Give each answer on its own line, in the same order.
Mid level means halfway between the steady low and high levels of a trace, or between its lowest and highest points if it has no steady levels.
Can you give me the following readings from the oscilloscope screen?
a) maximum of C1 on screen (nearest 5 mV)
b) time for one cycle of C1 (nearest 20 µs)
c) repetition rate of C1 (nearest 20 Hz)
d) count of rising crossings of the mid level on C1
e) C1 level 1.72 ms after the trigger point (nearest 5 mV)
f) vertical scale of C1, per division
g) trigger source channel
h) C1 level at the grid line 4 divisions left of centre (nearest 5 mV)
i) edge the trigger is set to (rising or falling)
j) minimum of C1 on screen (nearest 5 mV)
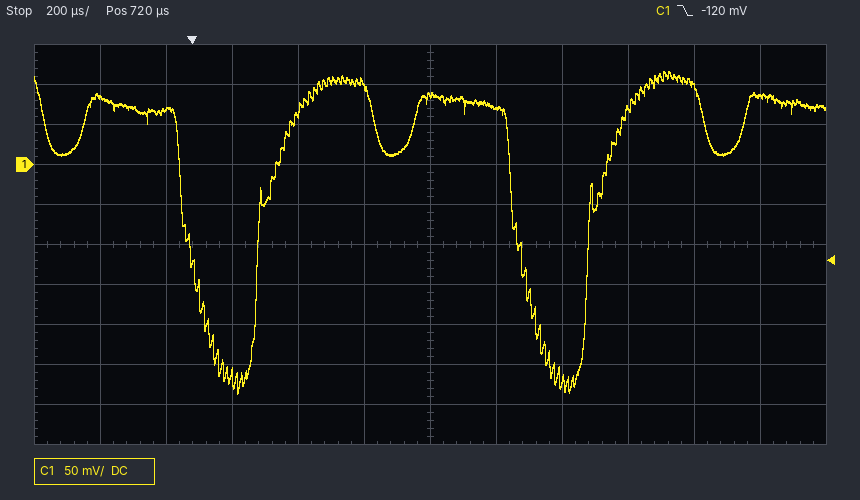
115 mV
1.00 ms
1.00 kHz
2
85 mV
50 mV
C1
70 mV
falling
-285 mV
